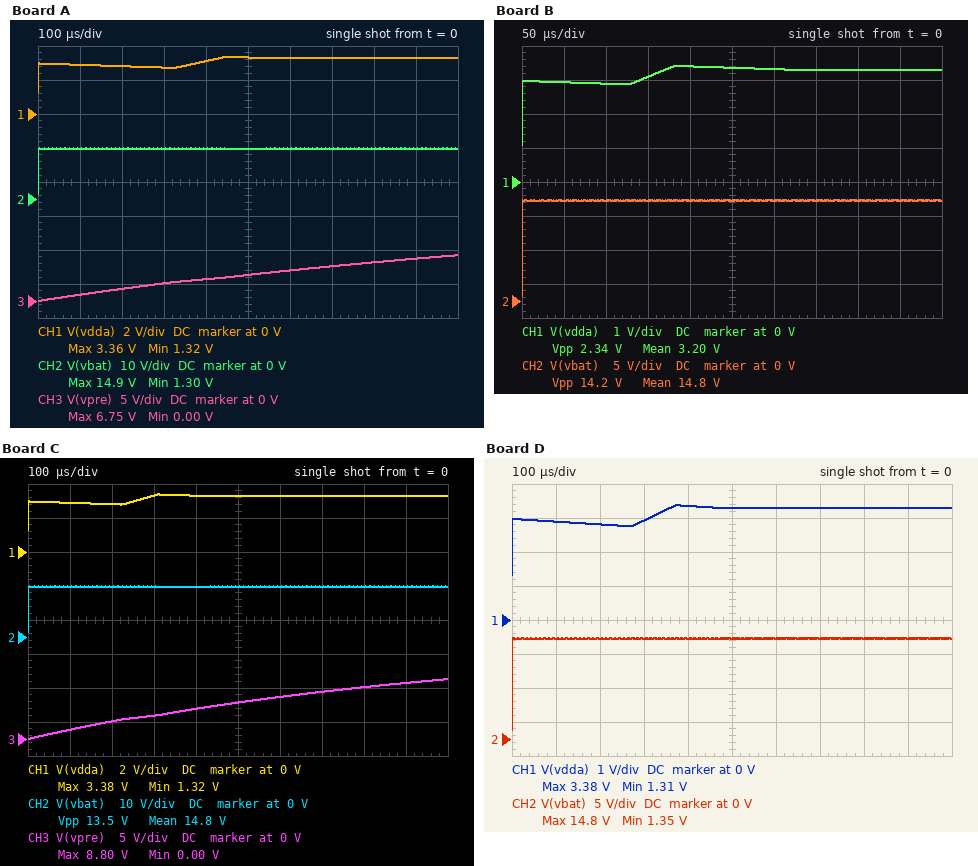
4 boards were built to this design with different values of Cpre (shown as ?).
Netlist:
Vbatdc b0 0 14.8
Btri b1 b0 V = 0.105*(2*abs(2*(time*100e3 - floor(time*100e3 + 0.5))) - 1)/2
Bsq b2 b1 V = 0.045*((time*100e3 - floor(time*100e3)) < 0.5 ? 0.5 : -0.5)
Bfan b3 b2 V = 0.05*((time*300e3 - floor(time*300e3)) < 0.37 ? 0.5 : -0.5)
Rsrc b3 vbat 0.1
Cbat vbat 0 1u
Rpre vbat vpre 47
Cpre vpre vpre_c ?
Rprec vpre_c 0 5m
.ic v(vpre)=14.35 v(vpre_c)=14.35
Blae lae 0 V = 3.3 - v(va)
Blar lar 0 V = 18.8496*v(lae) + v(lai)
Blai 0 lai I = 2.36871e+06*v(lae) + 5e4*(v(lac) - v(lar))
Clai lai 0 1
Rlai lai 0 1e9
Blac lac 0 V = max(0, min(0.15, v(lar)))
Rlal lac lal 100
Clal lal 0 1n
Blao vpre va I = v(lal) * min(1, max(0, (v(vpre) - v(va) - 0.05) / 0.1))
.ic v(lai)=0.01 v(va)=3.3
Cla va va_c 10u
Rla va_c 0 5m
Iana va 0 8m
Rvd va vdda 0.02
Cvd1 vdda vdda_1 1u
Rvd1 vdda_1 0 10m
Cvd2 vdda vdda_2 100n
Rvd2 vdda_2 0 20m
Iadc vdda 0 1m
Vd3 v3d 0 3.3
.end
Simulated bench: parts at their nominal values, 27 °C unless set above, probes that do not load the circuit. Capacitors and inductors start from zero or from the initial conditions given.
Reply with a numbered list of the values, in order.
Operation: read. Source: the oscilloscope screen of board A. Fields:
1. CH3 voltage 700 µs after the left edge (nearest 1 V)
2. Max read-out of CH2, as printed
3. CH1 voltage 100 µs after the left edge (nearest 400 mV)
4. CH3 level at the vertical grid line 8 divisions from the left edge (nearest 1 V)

1. 5 V
2. 14.9 V
3. 2.8 V
4. 6 V
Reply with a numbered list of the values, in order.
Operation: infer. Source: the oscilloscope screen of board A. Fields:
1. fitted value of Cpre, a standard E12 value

1. 33 µF
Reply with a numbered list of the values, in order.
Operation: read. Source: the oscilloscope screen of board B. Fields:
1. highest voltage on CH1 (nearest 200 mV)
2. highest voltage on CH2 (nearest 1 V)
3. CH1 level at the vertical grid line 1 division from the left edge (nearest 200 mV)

1. 3.4 V
2. 15 V
3. 3.0 V
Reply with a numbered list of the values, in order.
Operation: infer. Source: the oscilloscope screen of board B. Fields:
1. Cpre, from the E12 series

1. 12 µF
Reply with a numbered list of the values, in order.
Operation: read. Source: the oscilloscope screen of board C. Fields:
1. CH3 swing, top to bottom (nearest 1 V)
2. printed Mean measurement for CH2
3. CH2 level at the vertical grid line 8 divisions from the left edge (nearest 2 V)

1. 9 V
2. 14.8 V
3. 14 V
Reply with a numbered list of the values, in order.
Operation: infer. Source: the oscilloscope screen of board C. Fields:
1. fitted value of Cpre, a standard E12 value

1. 22 µF
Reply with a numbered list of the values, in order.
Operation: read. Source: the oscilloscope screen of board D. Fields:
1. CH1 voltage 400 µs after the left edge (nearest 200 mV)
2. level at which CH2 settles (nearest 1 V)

1. 3.4 V
2. 15 V
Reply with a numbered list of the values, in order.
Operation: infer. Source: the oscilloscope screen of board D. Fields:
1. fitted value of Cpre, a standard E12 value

1. 27 µF
